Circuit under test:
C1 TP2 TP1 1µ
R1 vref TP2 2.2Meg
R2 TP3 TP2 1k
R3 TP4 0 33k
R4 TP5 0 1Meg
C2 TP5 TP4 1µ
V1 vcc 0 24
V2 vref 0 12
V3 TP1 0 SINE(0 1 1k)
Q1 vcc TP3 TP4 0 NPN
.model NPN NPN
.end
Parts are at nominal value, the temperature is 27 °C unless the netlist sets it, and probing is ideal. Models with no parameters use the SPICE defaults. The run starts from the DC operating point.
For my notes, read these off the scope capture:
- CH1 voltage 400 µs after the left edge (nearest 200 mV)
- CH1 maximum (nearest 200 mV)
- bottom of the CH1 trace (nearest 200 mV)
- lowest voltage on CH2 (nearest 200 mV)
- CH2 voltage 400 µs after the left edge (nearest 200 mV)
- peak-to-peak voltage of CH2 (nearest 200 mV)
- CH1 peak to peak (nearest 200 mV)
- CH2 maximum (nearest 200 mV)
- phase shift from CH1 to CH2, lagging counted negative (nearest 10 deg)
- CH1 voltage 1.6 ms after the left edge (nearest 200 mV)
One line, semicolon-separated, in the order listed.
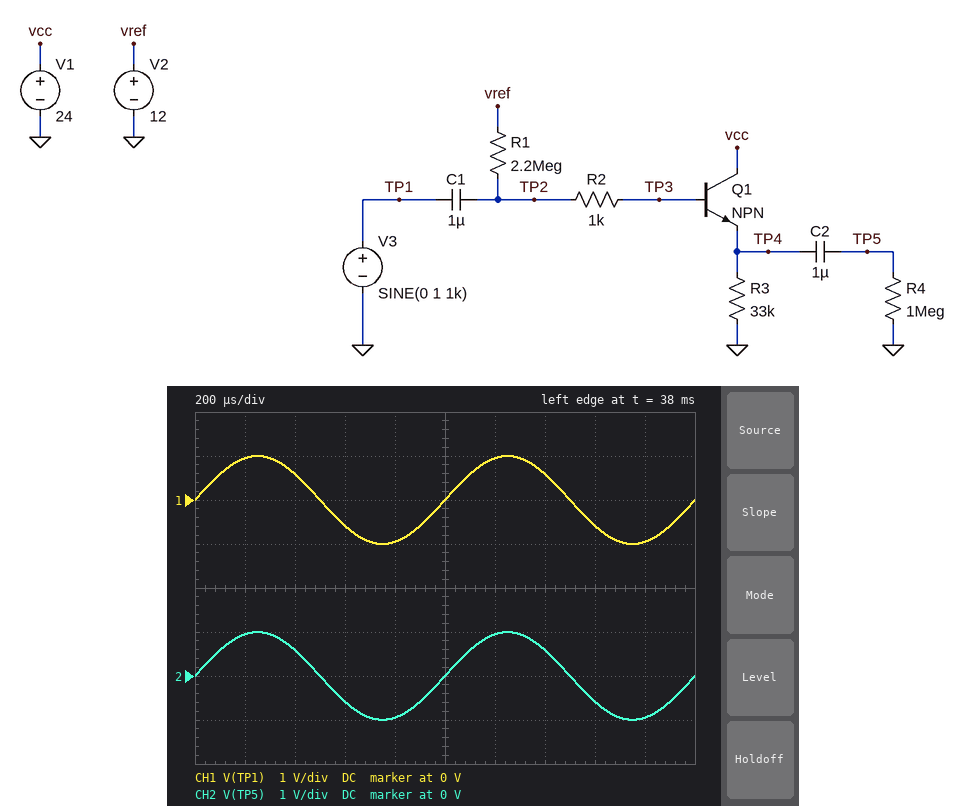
600 mV; 1.0 V; -1.0 V; -1.0 V; 600 mV; 2.0 V; 2.0 V; 1.0 V; 0 deg; -600 mV
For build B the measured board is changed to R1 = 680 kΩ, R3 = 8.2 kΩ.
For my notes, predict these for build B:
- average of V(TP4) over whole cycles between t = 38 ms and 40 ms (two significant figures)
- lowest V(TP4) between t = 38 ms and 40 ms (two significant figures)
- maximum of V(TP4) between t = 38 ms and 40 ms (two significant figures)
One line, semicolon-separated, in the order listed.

6.2 V; 5.2 V; 7.2 V
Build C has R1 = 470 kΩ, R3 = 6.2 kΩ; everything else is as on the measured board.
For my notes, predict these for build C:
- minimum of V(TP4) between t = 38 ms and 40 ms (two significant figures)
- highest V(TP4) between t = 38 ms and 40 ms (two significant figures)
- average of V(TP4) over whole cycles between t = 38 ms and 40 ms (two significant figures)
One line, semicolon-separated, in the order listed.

5.4 V; 7.4 V; 6.4 V
